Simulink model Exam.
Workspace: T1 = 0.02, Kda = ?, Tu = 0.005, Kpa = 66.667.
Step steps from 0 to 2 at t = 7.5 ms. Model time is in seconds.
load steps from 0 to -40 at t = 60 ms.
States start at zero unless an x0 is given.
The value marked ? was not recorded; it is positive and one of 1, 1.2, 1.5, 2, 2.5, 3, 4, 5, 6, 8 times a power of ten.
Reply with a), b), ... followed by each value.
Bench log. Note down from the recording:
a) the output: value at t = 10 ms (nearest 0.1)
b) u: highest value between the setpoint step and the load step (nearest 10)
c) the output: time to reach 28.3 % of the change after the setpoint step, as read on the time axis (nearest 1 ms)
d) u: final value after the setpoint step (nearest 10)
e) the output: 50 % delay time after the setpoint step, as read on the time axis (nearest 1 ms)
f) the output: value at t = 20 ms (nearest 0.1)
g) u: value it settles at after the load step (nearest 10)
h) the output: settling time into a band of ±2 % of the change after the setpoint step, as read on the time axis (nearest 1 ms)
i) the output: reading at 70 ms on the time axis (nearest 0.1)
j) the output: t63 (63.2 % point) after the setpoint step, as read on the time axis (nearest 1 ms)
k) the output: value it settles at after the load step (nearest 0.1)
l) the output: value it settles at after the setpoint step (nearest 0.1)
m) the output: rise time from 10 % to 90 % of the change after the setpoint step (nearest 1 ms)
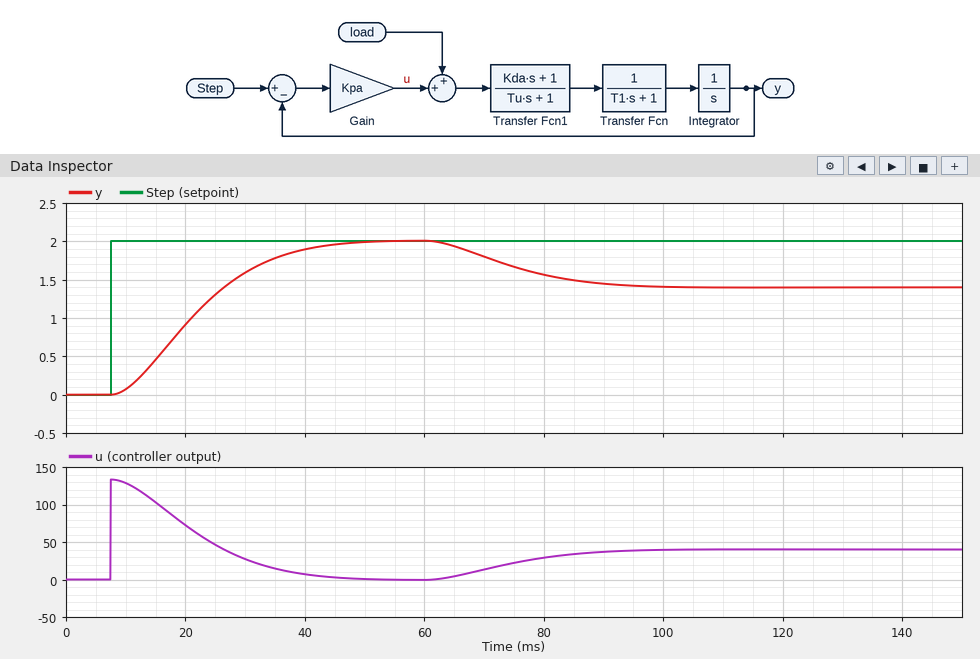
a) 0.1
b) 130
c) 16 ms
d) 0
e) 21 ms
f) 0.9
g) 40
h) 45 ms
i) 1.8
j) 24 ms
k) 1.4
l) 2.0
m) 24 ms
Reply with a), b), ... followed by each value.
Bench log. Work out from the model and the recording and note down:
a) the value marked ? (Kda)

a) 0.02
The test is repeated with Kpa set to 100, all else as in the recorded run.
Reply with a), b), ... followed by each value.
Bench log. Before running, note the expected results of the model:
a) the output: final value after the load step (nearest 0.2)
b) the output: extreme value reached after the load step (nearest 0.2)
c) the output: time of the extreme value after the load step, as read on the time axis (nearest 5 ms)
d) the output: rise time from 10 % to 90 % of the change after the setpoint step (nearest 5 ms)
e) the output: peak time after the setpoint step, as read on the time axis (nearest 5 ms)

a) 1.6
b) 1.6
c) 90 ms
d) 15 ms
e) 40 ms
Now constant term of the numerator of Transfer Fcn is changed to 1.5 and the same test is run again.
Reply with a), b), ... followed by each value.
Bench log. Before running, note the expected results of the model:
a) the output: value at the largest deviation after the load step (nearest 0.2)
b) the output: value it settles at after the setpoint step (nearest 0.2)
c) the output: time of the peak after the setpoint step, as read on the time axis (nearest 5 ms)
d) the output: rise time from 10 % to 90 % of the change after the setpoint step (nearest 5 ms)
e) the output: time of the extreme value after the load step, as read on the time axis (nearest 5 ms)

a) 1.4
b) 2.0
c) 40 ms
d) 15 ms
e) 90 ms
